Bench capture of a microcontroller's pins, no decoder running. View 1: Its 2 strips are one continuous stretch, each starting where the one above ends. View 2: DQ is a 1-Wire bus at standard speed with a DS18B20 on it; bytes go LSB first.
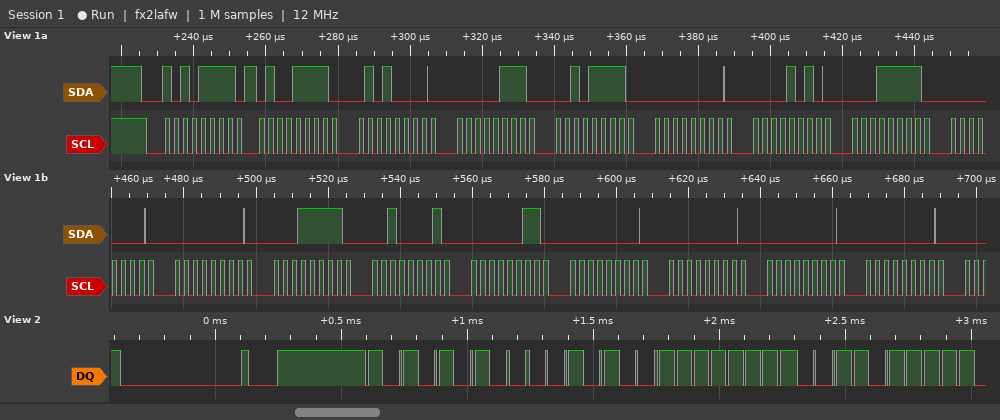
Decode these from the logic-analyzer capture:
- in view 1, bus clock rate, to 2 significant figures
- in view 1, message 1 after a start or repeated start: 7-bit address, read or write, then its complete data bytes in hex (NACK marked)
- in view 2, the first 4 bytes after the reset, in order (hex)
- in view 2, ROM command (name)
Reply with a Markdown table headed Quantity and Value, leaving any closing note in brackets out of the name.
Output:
| Quantity | Value |
|---|---|
| in view 1, bus clock rate, to 2 significant figures | 400 kHz |
| in view 1, message 1 after a start or repeated start: 7-bit address, read or write, then its complete data bytes in hex | 0x57 read: 4F 50 07 2F 00 0A 1F 00 00 1F 21 03 00 00 00 00 |
| in view 2, the first 4 bytes after the reset, in order | 55 28 FF EC |
| in view 2, ROM command | Match ROM |
